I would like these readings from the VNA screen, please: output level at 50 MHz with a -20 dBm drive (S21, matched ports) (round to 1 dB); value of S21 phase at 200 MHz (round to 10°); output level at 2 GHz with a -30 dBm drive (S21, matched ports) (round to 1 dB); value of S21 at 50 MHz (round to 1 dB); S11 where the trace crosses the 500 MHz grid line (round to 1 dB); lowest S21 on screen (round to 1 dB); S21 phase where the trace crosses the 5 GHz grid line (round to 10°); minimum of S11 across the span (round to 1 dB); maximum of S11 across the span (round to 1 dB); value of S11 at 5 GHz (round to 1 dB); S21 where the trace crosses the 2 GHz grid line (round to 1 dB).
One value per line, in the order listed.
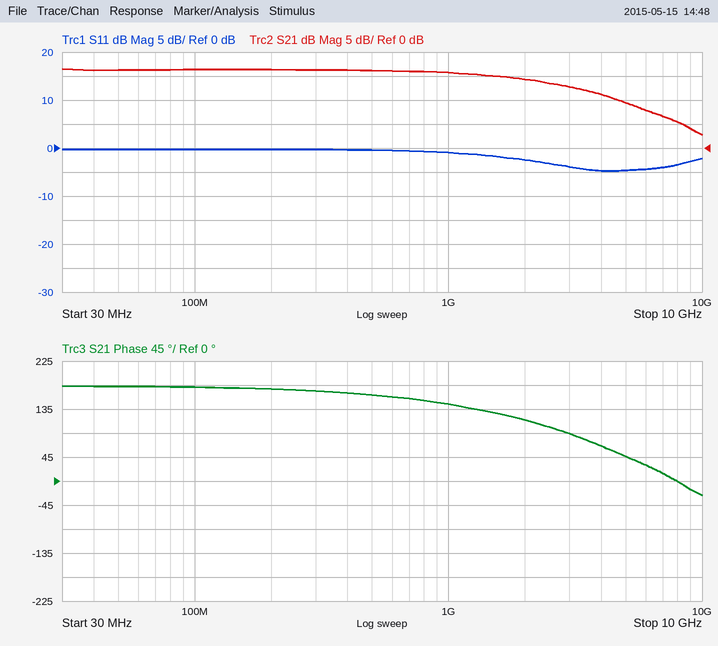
-4 dBm
170°
-16 dBm
16 dB
0 dB
3 dB
50°
-5 dB
0 dB
-5 dB
14 dB
